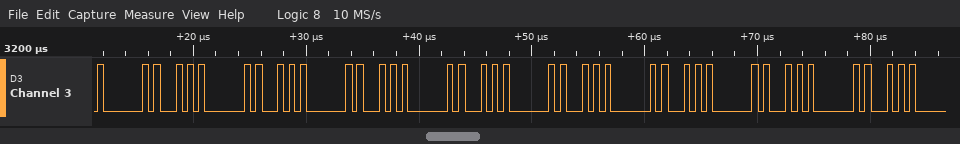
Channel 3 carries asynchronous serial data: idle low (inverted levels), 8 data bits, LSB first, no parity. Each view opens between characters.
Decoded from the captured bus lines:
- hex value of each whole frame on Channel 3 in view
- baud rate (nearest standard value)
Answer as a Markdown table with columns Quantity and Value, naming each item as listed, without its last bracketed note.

| Quantity | Value |
|---|---|
| hex value of each whole frame on Channel 3 in view | 7F, 57, 5D, 7F, 57, 5D, 7F, 57, 5D, 7F, 57, 5D |
| baud rate | 2000000 baud |
